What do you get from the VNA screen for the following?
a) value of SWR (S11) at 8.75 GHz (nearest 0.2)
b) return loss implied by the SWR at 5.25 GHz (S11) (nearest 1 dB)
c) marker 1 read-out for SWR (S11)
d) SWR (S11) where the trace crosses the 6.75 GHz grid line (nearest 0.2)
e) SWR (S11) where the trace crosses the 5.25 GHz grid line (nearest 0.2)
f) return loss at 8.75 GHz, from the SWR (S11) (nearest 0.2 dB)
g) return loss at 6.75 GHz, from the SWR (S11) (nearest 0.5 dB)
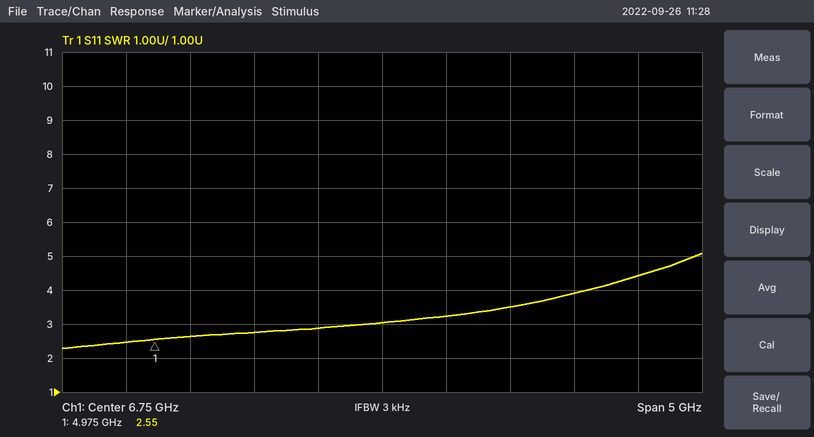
4.4
7 dB
2.55
3.0
2.6
4.0 dB
6.0 dB
